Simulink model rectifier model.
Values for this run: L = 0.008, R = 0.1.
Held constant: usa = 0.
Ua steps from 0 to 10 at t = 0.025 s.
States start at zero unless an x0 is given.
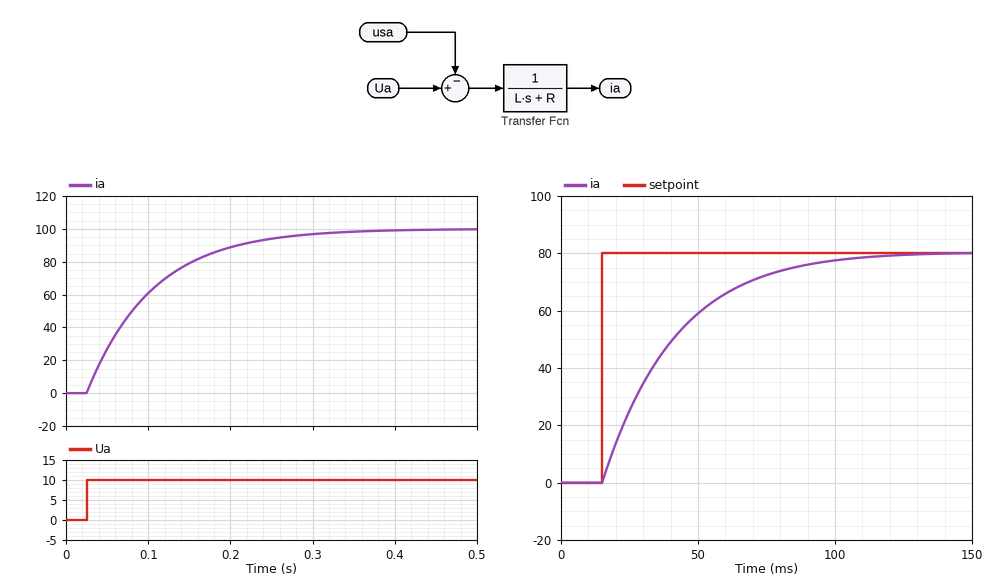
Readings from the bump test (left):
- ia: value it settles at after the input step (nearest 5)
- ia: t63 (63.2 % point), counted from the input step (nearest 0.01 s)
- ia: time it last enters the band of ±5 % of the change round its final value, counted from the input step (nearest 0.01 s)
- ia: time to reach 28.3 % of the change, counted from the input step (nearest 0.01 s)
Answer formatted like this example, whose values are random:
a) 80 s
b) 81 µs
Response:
a) 100
b) 0.08 s
c) 0.24 s
d) 0.03 s
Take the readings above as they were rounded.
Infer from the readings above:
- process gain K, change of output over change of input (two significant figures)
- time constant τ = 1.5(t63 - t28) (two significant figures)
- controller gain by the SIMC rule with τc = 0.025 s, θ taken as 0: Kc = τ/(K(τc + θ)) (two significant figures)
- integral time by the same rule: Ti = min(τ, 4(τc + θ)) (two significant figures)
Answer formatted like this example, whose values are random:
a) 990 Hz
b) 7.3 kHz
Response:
a) 10
b) 0.075 s
c) 0.30
d) 0.075 s
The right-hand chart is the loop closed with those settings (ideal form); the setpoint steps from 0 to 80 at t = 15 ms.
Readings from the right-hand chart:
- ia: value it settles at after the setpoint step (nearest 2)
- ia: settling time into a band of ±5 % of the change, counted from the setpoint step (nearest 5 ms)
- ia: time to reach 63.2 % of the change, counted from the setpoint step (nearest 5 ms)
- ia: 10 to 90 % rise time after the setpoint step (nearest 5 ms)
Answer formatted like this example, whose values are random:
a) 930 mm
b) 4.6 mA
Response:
a) 80
b) 75 ms
c) 25 ms
d) 55 ms
